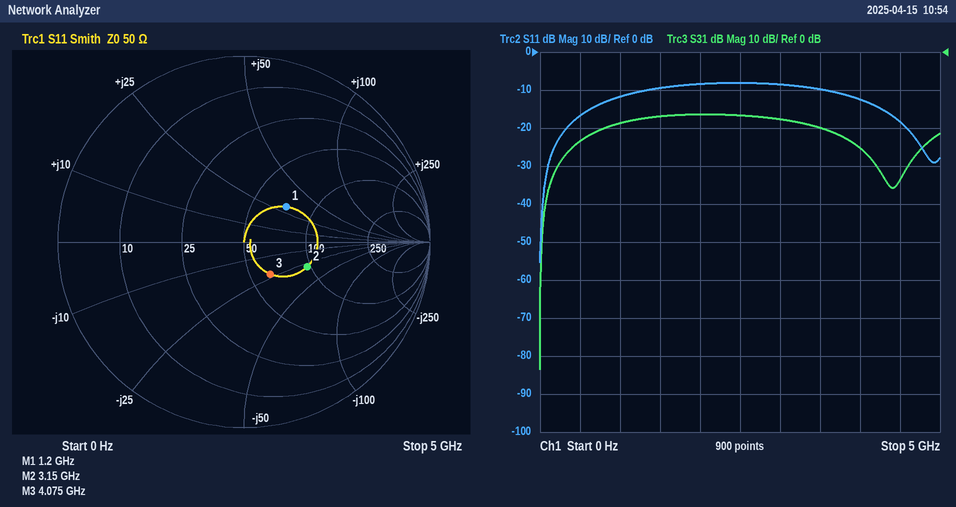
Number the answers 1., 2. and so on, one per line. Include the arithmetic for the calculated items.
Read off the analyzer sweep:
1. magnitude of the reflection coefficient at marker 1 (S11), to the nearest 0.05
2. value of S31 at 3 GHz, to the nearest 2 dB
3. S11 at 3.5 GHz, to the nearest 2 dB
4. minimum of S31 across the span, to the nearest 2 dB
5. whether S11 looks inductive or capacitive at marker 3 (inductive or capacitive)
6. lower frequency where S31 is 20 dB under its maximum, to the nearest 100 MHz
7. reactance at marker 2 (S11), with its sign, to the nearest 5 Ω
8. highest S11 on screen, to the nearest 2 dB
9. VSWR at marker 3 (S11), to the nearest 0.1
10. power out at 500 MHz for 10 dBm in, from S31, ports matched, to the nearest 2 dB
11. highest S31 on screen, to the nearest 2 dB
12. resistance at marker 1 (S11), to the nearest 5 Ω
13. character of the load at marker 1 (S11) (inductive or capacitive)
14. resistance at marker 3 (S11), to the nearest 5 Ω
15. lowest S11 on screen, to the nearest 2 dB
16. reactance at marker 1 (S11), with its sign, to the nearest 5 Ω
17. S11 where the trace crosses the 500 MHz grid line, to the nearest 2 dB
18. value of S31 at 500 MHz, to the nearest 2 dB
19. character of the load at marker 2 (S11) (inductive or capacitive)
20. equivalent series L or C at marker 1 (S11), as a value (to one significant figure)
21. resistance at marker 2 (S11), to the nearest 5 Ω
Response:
1. 0.30
2. -18 dB
3. -10 dB
4. -84 dB
5. capacitive
6. 100 MHz
7. -30 Ω
8. -8 dB
9. 1.6
10. 10 dBm + (-24 dB) = -14 dBm
11. -16 dB
12. 70 Ω
13. inductive
14. 60 Ω
15. -56 dB
16. +30 Ω
17. -16 dB
18. -24 dB
19. capacitive
20. L = 30 Ω/(2π × 1.2 GHz) ≈ 4 nH
21. 95 Ω
